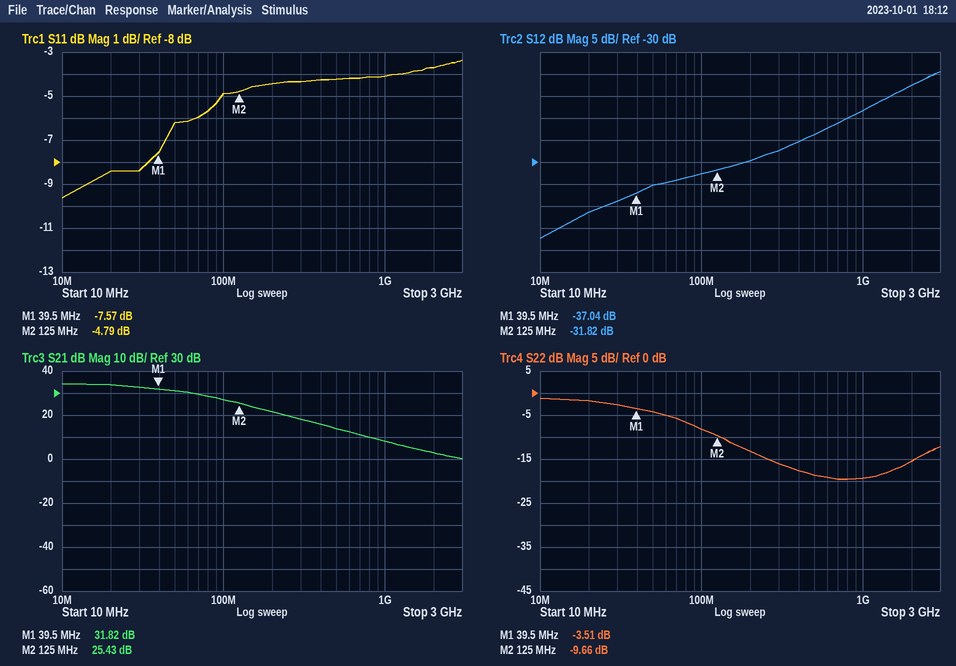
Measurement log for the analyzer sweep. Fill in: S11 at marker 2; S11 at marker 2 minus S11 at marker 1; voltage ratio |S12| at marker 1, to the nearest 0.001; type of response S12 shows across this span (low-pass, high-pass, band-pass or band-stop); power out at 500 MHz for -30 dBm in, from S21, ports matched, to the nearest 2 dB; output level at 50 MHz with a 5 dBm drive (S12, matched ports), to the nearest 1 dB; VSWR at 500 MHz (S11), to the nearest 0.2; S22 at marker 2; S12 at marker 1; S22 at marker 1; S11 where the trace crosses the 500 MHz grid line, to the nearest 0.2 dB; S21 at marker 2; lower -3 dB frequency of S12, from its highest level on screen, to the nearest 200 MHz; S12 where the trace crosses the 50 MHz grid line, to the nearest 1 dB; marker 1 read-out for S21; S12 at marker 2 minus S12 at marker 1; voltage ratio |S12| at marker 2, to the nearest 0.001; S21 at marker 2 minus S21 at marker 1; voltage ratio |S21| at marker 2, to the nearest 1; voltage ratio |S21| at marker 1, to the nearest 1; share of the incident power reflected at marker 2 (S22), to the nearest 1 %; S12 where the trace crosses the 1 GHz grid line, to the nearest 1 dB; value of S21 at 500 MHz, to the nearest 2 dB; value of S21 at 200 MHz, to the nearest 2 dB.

-4.79 dB
2.78 dB
0.014
high-pass
-16 dBm
-30 dBm
4.2
-9.66 dB
-37.04 dB
-3.51 dB
-4.2 dB
25.43 dB
2.0 GHz
-35 dB
31.82 dB
5.22 dB
0.026
-6.39 dB
19
39
11 %
-18 dB
14 dB
22 dB
